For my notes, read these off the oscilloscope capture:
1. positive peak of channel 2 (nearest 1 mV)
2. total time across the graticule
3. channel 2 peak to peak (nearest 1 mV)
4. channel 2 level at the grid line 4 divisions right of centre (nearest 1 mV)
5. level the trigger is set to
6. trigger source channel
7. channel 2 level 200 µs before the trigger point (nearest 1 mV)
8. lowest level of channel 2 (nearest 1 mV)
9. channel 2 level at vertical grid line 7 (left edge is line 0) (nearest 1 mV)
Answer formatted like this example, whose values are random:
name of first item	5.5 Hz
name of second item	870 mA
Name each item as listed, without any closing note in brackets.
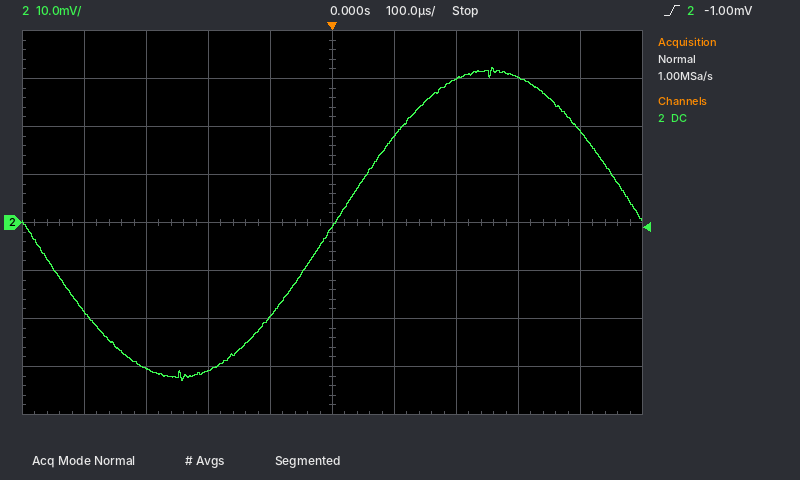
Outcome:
positive peak of channel 2	32 mV
total time across the graticule	1 ms
channel 2 peak to peak	65 mV
channel 2 level at the grid line 4 divisions right of centre	19 mV
level the trigger is set to	-1.00 mV
trigger source channel	channel 2
channel 2 level 200 µs before the trigger point	-31 mV
lowest level of channel 2	-33 mV
channel 2 level at vertical grid line 7 (left edge is line 0)	30 mV
